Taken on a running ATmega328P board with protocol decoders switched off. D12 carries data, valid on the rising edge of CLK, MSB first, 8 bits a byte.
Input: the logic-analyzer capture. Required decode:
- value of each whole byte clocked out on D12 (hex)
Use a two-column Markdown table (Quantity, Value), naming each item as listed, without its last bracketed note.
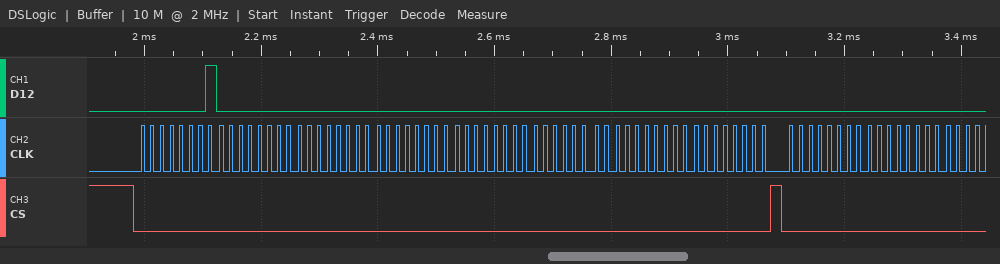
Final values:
| Quantity | Value |
|---|---|
| value of each whole byte clocked out on D12 | 0x01 0x00 0x00 0x00 0x00 0x00 0x00 0x00 0x00 0x00 |
